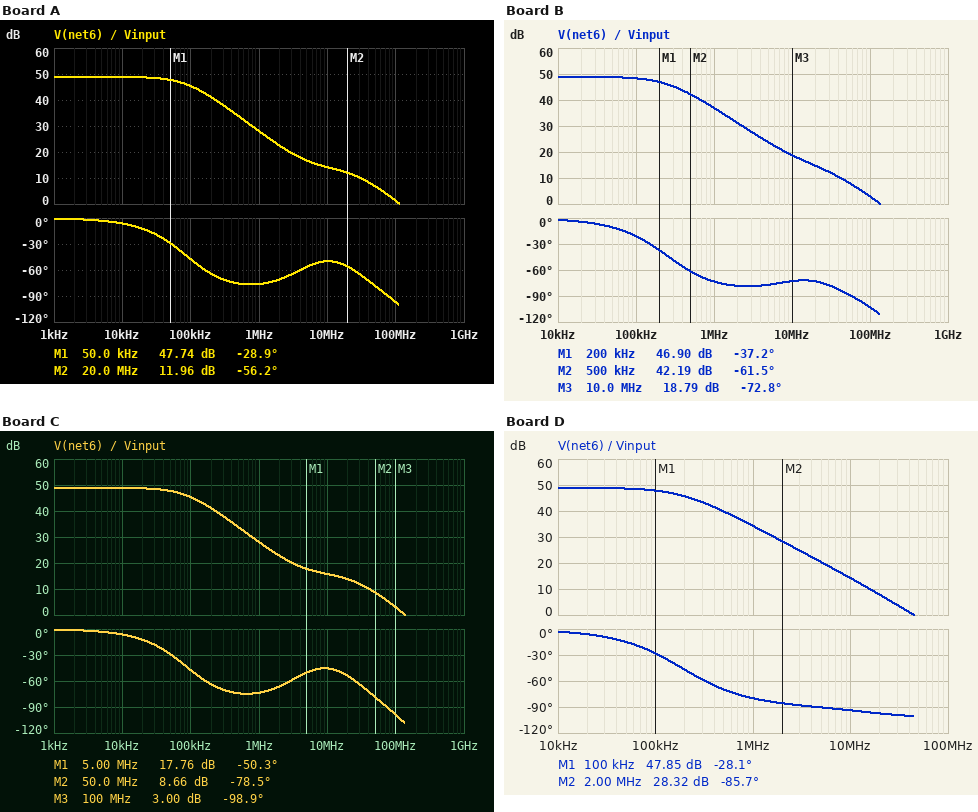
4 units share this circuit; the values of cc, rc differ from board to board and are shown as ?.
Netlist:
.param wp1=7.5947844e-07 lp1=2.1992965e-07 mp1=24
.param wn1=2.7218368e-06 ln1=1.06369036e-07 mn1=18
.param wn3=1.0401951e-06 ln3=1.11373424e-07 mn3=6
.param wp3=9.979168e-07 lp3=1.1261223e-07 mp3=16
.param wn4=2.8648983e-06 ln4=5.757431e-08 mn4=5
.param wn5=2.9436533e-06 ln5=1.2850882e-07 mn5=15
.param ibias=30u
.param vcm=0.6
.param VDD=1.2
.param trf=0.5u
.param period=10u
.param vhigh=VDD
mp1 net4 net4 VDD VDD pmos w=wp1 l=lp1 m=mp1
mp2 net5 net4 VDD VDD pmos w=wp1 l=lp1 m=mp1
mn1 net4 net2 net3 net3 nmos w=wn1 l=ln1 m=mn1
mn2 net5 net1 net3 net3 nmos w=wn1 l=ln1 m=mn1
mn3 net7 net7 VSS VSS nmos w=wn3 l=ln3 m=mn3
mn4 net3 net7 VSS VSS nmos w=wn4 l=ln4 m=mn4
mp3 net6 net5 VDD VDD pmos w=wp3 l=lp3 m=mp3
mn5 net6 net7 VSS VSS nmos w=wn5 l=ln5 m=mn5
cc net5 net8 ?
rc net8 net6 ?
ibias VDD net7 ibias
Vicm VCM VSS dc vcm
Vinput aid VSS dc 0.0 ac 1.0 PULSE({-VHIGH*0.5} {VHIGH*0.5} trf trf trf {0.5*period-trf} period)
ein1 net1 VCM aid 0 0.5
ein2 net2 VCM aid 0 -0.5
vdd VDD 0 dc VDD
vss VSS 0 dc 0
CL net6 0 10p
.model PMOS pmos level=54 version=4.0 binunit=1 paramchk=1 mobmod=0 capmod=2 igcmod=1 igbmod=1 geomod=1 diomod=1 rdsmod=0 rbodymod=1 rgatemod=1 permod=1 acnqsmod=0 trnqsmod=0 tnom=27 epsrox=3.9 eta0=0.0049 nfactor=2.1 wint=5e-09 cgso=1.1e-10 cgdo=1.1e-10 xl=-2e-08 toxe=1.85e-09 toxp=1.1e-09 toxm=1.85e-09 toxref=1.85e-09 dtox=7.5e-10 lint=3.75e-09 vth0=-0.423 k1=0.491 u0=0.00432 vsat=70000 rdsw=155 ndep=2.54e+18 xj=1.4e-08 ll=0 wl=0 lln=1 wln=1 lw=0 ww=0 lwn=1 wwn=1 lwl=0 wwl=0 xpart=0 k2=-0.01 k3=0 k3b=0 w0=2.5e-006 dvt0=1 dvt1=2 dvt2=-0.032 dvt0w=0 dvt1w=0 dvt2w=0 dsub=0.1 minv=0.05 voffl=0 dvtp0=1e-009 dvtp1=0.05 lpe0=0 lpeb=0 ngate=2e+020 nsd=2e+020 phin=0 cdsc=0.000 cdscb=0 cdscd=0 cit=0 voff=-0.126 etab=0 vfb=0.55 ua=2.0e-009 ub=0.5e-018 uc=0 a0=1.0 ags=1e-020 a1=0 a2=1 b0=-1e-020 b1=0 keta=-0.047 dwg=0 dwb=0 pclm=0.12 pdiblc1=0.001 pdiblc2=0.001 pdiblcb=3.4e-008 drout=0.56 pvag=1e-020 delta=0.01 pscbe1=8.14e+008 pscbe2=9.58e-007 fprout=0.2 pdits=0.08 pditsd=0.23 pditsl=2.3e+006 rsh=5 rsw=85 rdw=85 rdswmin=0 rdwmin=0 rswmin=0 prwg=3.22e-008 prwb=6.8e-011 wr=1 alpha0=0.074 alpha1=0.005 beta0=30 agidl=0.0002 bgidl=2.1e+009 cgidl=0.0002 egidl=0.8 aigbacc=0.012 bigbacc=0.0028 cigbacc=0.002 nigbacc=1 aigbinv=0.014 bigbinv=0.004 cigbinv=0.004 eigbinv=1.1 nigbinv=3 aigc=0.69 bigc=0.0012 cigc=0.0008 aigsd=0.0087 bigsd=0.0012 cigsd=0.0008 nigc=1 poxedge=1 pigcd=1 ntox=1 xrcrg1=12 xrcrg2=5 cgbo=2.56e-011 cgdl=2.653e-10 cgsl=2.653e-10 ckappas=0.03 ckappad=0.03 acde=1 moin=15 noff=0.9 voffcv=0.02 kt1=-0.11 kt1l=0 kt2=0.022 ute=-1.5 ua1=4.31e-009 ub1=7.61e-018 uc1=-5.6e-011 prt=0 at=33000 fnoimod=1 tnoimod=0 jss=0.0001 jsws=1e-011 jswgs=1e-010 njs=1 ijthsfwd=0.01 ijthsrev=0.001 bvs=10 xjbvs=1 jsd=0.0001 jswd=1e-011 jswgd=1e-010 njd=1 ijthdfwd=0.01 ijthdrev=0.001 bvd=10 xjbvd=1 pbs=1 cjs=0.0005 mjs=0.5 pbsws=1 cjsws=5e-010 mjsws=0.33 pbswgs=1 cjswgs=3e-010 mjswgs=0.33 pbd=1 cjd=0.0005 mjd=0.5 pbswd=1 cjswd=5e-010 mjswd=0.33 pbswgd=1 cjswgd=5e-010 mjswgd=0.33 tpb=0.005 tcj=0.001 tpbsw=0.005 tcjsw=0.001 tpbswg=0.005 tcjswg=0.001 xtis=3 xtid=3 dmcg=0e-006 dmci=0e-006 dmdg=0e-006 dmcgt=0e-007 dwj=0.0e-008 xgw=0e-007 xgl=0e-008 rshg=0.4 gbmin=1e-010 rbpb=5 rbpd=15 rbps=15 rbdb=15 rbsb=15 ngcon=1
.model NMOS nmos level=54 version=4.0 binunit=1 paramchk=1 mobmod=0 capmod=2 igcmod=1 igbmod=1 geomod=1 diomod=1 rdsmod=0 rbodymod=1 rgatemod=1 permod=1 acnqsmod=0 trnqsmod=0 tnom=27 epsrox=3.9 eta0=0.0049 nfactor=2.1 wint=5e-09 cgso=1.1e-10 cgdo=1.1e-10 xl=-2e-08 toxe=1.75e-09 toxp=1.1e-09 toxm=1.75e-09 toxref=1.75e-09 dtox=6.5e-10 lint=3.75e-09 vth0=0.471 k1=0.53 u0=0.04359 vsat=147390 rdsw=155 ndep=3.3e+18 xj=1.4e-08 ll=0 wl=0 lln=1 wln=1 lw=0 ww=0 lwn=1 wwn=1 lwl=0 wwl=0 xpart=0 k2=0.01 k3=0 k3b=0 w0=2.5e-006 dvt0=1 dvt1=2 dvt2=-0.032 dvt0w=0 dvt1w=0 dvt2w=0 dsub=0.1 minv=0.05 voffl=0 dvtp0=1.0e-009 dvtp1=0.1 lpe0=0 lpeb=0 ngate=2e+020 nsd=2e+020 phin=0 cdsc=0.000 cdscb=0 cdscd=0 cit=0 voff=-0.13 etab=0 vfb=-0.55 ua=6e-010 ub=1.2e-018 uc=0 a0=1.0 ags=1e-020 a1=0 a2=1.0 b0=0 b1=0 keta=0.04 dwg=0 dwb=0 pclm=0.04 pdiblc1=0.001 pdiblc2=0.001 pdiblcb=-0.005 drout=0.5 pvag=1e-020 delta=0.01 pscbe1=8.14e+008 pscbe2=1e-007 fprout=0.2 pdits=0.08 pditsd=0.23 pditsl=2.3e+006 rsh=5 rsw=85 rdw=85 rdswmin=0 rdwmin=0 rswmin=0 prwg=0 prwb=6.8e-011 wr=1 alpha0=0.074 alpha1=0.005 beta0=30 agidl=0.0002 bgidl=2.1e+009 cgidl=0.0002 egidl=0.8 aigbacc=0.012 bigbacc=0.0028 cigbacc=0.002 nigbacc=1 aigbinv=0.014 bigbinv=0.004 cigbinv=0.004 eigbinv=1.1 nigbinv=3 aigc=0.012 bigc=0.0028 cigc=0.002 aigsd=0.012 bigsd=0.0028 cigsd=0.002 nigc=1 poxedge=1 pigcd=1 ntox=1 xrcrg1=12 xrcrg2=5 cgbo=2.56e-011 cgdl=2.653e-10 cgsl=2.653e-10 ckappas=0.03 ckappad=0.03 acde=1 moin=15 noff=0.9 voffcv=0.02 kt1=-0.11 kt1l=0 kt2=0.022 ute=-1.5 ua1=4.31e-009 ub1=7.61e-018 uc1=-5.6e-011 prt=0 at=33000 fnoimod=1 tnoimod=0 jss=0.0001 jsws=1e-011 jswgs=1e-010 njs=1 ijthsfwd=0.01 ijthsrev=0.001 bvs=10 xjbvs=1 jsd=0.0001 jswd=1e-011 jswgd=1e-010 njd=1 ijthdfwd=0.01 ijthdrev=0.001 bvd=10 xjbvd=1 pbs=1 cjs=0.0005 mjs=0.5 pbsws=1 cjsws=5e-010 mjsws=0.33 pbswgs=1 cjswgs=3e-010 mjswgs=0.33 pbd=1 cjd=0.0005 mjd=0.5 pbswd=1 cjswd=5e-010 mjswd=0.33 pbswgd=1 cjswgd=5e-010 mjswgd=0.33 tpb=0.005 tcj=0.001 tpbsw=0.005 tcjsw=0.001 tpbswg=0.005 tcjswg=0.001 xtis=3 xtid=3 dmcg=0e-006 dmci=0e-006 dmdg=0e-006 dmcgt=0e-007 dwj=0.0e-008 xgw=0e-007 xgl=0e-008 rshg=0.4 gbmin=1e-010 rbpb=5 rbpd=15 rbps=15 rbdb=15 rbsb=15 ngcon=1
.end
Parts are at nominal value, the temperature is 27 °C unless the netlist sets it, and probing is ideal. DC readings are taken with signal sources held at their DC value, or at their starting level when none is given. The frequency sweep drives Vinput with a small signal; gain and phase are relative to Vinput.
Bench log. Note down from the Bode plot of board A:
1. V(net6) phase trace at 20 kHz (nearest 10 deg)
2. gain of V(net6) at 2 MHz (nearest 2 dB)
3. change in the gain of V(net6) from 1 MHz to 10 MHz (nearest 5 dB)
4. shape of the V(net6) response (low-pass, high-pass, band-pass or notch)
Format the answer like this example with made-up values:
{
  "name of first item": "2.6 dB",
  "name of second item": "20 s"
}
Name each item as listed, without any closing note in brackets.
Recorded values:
{
  "V(net6) phase trace at 20 kHz": "-10 deg",
  "gain of V(net6) at 2 MHz": "22 dB",
  "change in the gain of V(net6) from 1 MHz to 10 MHz": "-15 dB",
  "shape of the V(net6) response": "low-pass"
}
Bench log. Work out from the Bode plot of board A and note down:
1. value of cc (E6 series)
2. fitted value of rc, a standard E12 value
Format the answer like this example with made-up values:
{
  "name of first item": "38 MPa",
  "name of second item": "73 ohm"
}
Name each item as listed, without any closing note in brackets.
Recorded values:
{
  "value of cc": "10 pF",
  "fitted value of rc, a standard E12 value": "3.9 kΩ"
}
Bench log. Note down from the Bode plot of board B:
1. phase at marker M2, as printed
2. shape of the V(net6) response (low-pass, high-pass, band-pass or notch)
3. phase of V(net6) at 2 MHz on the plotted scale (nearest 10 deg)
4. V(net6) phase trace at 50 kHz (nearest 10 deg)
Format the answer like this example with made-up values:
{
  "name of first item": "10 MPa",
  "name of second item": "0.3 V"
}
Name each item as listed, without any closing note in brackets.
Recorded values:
{
  "phase at marker M2, as printed": "-61.5 deg",
  "shape of the V(net6) response": "low-pass",
  "phase of V(net6) at 2 MHz on the plotted scale": "-80 deg",
  "V(net6) phase trace at 50 kHz": "-10 deg"
}
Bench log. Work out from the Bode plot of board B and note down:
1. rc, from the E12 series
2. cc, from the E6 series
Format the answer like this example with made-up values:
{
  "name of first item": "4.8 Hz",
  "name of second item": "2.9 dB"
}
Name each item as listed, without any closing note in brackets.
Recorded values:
{
  "rc, from the E12 series": "4.7 kΩ",
  "cc, from the E6 series": "3.3 pF"
}
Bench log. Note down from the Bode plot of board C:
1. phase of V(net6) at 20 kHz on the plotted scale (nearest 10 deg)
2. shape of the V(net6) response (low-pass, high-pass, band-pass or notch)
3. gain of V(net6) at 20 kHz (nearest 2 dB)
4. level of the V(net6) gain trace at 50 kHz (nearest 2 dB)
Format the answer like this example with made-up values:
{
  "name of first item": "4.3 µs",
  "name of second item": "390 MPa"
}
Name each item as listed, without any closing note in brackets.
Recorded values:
{
  "phase of V(net6) at 20 kHz on the plotted scale": "-10 deg",
  "shape of the V(net6) response": "low-pass",
  "gain of V(net6) at 20 kHz": "48 dB",
  "level of the V(net6) gain trace at 50 kHz": "48 dB"
}
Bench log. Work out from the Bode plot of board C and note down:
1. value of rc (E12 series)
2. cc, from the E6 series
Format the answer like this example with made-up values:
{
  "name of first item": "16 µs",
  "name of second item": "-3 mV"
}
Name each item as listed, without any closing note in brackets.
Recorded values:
{
  "value of rc": "4.7 kΩ",
  "cc, from the E6 series": "10 pF"
}
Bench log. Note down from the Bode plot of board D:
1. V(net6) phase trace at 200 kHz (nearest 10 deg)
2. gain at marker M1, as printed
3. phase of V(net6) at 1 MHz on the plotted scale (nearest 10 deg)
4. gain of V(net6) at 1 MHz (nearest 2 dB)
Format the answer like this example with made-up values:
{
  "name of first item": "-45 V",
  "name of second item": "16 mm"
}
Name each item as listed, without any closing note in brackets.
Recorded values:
{
  "V(net6) phase trace at 200 kHz": "-50 deg",
  "gain at marker M1, as printed": "47.85 dB",
  "phase of V(net6) at 1 MHz on the plotted scale": "-80 deg",
  "gain of V(net6) at 1 MHz": "34 dB"
}
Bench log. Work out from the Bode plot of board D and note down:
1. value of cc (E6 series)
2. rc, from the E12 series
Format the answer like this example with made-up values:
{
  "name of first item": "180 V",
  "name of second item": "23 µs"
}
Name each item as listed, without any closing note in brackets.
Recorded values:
{
  "value of cc": "4.7 pF",
  "rc, from the E12 series": "1.8 kΩ"
}
